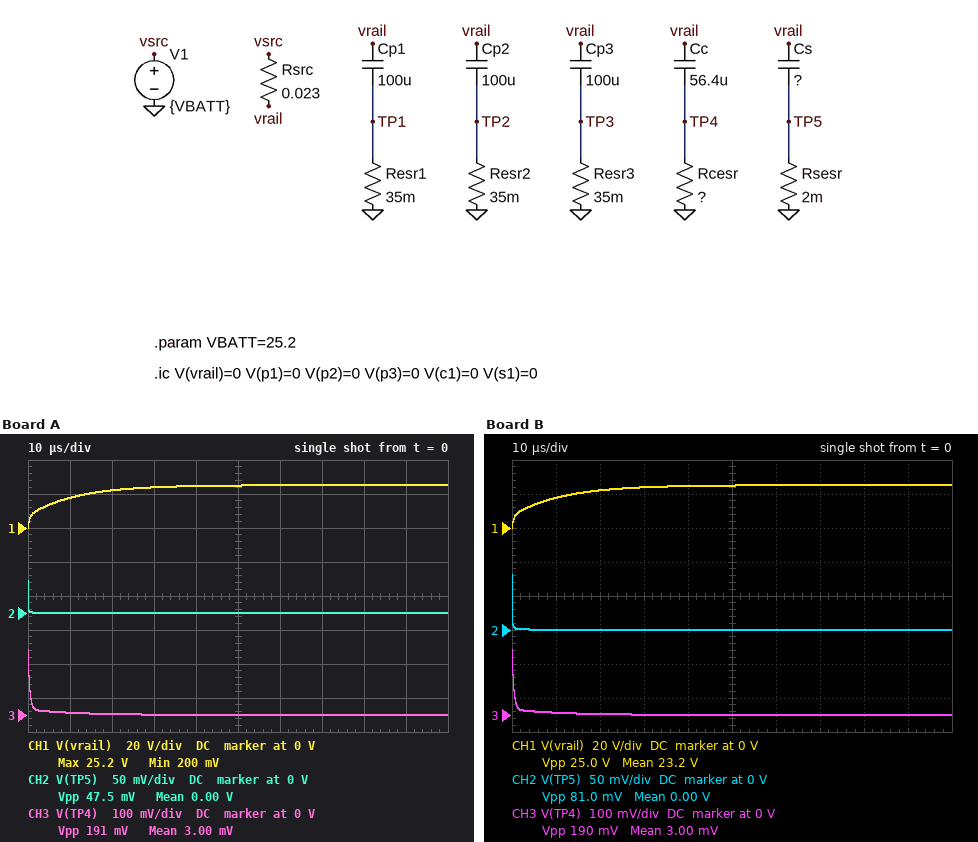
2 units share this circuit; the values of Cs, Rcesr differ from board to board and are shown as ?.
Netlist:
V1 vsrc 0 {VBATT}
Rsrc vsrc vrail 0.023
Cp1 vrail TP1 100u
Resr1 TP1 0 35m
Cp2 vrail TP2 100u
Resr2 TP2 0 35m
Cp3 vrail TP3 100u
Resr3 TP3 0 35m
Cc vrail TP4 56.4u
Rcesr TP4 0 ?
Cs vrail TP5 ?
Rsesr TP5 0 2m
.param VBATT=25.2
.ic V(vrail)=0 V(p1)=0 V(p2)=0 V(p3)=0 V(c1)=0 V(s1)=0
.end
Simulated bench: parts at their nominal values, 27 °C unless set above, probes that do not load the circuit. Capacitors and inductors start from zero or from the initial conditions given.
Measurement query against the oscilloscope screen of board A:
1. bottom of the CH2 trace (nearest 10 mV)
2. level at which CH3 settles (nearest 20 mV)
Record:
0 V
0 V
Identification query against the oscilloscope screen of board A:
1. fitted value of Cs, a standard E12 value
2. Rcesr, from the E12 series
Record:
150 nF
180 µΩ
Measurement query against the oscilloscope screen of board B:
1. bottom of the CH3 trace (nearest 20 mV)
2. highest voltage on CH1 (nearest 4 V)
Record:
0 V
24 V
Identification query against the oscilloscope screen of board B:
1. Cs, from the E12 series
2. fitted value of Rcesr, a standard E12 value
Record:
330 nF
180 µΩ
